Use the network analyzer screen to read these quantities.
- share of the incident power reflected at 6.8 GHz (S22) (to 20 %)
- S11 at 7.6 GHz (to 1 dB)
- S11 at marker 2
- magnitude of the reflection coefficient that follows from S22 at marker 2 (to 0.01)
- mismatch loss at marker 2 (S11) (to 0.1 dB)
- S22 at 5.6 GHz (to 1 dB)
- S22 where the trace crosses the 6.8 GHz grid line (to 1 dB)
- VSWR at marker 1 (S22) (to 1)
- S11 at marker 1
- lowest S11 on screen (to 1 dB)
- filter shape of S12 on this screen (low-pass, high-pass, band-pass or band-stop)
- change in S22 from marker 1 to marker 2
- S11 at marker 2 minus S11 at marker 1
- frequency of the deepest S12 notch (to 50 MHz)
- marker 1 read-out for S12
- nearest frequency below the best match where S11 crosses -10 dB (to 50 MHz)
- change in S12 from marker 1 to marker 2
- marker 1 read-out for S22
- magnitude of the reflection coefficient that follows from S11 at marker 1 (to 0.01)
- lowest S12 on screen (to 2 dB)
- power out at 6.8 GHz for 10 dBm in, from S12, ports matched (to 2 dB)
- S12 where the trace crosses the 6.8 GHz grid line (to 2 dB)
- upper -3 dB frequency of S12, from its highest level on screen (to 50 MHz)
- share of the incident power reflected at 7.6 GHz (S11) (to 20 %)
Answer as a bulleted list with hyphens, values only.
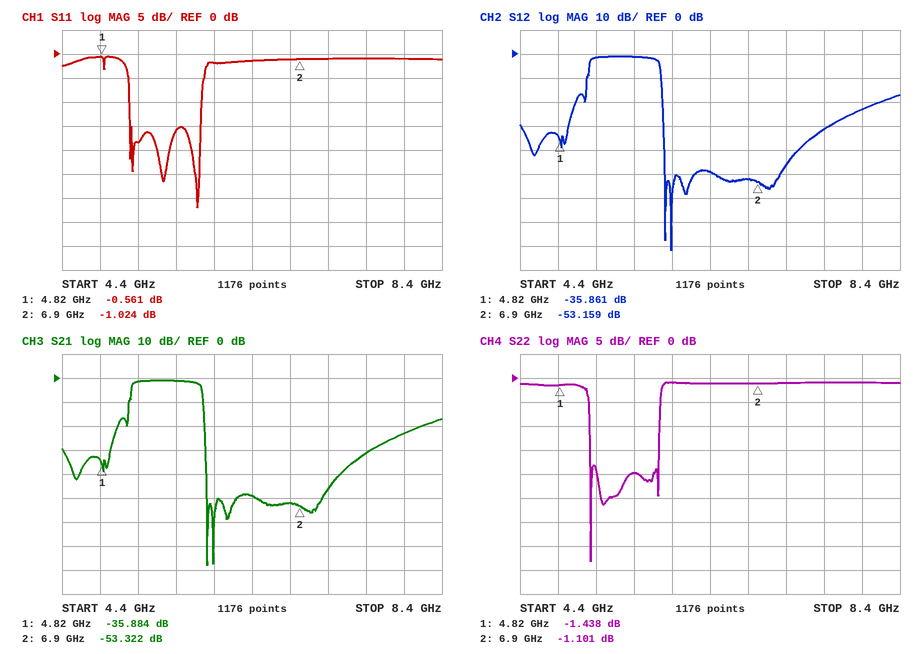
- 80 %
- -1 dB
- -1.024 dB
- 0.88
- 6.8 dB
- -20 dB
- -1 dB
- 12
- -0.561 dB
- -32 dB
- band-pass
- 0.337 dB
- -0.463 dB
- 6.00 GHz
- -35.861 dB
- 5.10 GHz
- -17.298 dB
- -1.438 dB
- 0.94
- -82 dB
- -42 dBm
- -52 dB
- 5.85 GHz
- 80 %
